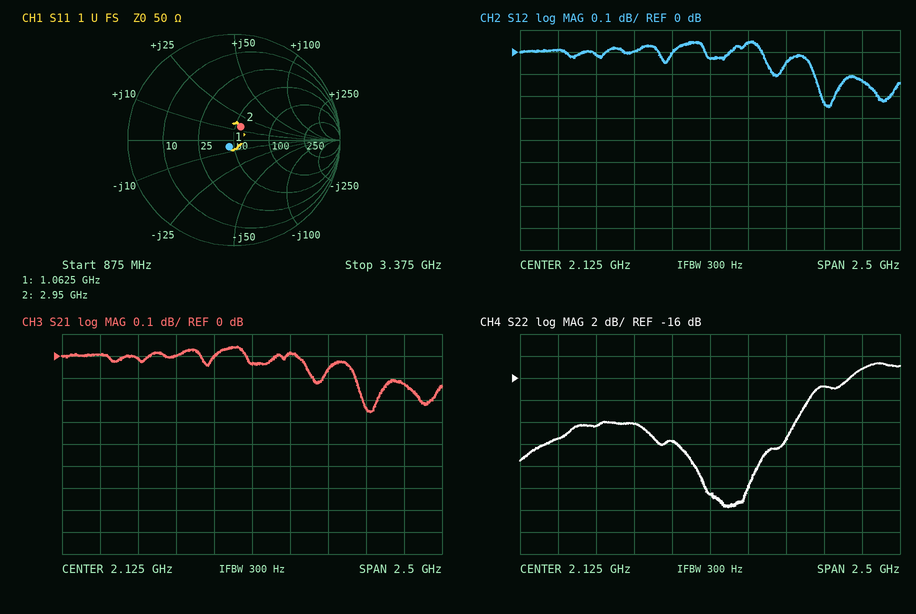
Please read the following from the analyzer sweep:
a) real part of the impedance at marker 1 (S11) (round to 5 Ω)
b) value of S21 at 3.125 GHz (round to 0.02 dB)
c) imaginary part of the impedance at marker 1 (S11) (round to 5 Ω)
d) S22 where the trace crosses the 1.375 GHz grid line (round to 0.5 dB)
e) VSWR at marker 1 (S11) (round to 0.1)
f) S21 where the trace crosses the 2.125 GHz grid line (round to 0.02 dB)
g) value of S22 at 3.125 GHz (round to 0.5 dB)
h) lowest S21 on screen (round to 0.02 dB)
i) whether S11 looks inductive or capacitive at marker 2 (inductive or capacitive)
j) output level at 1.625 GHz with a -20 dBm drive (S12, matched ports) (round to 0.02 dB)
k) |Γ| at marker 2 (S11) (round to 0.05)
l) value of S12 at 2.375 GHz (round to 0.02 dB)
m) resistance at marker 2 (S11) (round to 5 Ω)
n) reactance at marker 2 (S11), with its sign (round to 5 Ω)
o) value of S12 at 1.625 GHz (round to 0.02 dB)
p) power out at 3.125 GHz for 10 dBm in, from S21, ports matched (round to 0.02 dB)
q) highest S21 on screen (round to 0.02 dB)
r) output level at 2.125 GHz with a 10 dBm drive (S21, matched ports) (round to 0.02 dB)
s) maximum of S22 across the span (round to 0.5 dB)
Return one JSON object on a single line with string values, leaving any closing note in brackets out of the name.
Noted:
{"real part of the impedance at marker 1 (S11)": "45 Ω", "value of S21 at 3.125 GHz": "-0.12 dB", "imaginary part of the impedance at marker 1 (S11)": "-5 Ω", "S22 where the trace crosses the 1.375 GHz grid line": "-20.5 dB", "VSWR at marker 1 (S11)": "1.2", "S21 where the trace crosses the 2.125 GHz grid line": "-0.04 dB", "value of S22 at 3.125 GHz": "-15.0 dB", "lowest S21 on screen": "-0.26 dB", "whether S11 looks inductive or capacitive at marker 2": "inductive", "output level at 1.625 GHz with a -20 dBm drive (S12, matched ports)": "-20.00 dBm", "|Γ| at marker 2 (S11)": "0.15", "value of S12 at 2.375 GHz": "0.04 dB", "resistance at marker 2 (S11)": "55 Ω", "reactance at marker 2 (S11), with its sign": "+15 Ω", "value of S12 at 1.625 GHz": "0.00 dB", "power out at 3.125 GHz for 10 dBm in, from S21, ports matched": "9.88 dBm", "highest S21 on screen": "0.04 dB", "output level at 2.125 GHz with a 10 dBm drive (S21, matched ports)": "9.96 dBm", "maximum of S22 across the span": "-14.5 dB"}
